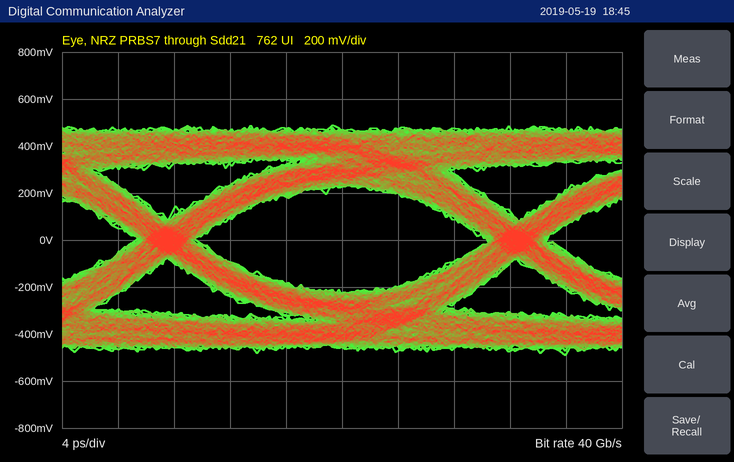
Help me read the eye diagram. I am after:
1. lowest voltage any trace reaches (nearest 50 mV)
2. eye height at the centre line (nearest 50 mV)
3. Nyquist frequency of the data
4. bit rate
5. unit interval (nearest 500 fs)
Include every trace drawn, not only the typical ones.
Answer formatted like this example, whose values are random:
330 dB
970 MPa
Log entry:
-500 mV
450 mV
20 GHz
40 Gb/s
25.0 ps
